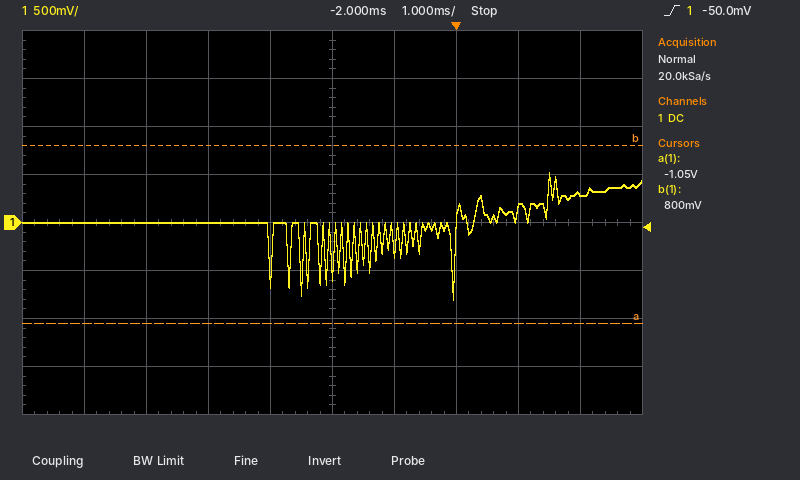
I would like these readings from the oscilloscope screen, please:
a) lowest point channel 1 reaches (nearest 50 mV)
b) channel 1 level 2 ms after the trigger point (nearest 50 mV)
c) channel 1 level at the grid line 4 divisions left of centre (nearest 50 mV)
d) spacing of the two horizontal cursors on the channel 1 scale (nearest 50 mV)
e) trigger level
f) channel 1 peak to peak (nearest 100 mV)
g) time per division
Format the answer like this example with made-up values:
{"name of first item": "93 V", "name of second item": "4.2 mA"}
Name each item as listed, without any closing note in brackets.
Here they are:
{"lowest point channel 1 reaches": "-800 mV", "channel 1 level 2 ms after the trigger point": "300 mV", "channel 1 level at the grid line 4 divisions left of centre": "0 mV", "spacing of the two horizontal cursors on the channel 1 scale": "1.85 V", "trigger level": "-50.0 mV", "channel 1 peak to peak": "1.30 V", "time per division": "1 ms"}
